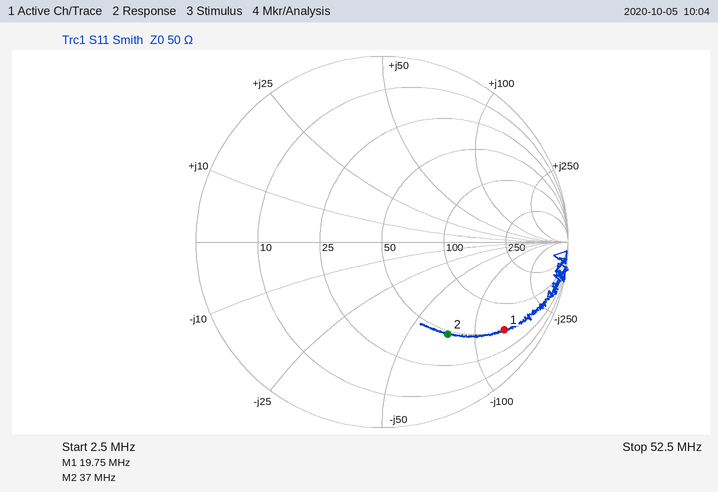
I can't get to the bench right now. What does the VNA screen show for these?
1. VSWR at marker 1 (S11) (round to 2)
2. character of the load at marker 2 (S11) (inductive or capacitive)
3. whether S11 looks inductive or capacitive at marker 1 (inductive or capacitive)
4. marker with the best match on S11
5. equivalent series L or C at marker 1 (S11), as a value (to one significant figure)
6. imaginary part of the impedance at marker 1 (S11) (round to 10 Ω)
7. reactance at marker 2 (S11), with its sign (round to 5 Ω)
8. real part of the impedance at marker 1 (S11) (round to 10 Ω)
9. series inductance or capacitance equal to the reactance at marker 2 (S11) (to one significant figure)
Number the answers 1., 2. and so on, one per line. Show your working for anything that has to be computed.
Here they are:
1. 10
2. capacitive
3. capacitive
4. marker 2
5. C = 1/(2π × 19.75 MHz × 140 Ω) ≈ 57.6 pF, so 60 pF to one significant figure
6. -140 Ω
7. -75 Ω
8. 50 Ω
9. C = 1/(2π × 37 MHz × 75 Ω) ≈ 57.4 pF, so 60 pF to one significant figure
